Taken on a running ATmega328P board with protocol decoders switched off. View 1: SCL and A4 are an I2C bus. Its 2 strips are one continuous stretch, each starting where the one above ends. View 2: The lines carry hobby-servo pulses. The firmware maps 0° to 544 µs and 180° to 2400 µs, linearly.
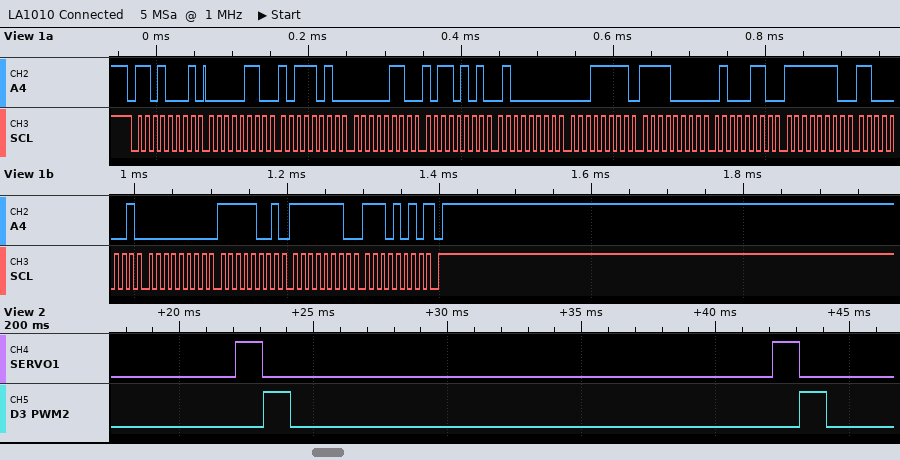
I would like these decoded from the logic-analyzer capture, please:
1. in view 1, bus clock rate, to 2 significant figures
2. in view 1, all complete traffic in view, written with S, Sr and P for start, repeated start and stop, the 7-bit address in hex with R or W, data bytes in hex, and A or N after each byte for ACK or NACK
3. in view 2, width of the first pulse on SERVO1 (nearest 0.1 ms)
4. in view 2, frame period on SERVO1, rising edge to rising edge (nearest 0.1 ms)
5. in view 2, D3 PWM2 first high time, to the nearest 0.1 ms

100 kHz
S 68R A 06 A BA A 06 A B5 A 40 A 1F A F0 A 46 A FE A C1 A 00 A F9 A FE A EA N P
1.0 ms
20.0 ms
1.0 ms
